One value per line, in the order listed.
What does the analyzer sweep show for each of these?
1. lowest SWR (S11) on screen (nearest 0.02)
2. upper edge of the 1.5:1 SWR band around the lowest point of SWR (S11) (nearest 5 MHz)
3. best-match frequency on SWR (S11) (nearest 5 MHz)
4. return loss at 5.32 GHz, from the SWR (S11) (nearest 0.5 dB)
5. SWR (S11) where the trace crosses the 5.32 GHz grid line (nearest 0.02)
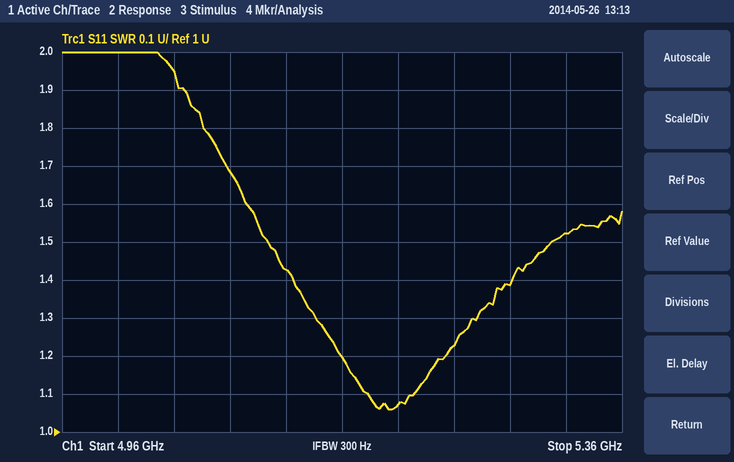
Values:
1.06
5.310 GHz
5.195 GHz
13.5 dB
1.52
